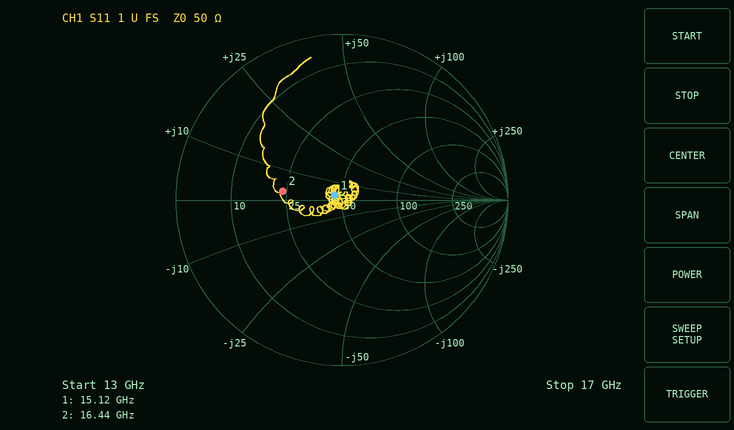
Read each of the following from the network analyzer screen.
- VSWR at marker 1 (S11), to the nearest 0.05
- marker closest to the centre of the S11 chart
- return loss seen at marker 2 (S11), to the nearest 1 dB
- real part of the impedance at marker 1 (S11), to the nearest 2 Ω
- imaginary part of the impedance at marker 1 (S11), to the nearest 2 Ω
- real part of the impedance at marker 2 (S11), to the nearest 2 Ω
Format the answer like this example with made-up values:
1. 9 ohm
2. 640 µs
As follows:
1. 1.10
2. marker 1
3. 9 dB
4. 46 Ω
5. +2 Ω
6. 24 Ω
